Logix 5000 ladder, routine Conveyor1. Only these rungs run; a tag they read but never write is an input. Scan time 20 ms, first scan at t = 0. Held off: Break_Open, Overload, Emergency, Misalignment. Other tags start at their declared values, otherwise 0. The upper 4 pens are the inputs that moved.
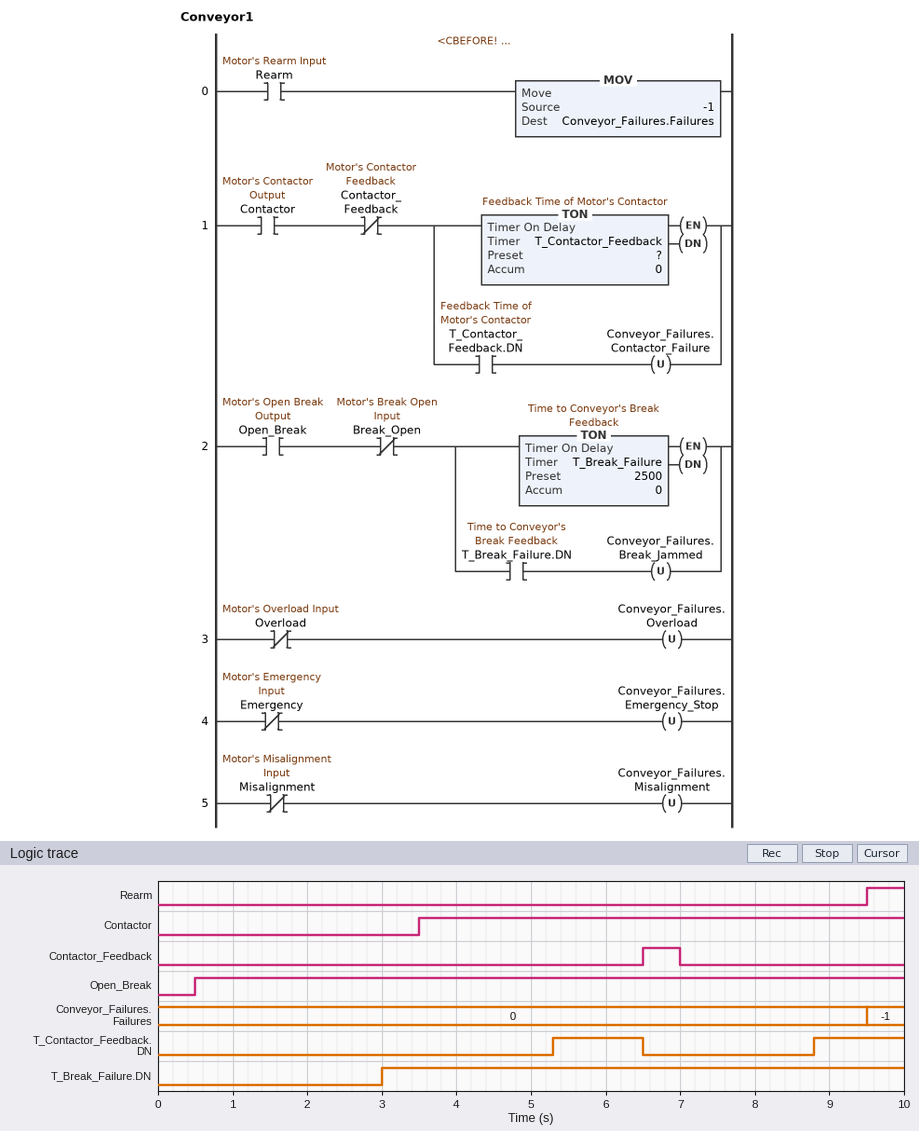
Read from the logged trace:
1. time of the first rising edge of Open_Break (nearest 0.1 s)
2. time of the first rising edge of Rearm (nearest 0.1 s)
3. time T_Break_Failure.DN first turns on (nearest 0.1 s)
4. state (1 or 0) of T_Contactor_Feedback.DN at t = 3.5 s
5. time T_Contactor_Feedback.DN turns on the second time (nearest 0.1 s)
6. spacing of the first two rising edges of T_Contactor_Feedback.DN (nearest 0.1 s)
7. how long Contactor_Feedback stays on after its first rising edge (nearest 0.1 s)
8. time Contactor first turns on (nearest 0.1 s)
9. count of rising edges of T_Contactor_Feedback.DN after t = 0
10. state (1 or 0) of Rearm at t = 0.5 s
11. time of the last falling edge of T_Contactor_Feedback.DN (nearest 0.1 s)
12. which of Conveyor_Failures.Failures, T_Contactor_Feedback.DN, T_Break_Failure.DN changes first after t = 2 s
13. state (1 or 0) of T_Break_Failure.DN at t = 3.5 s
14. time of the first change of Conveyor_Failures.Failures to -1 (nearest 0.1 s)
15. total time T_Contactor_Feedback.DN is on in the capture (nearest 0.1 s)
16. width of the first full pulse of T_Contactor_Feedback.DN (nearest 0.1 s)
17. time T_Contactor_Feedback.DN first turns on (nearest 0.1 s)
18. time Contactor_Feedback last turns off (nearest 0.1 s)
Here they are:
0.5 s
9.5 s
3.0 s
0
8.8 s
3.5 s
0.5 s
3.5 s
2
0
6.5 s
T_Break_Failure.DN
1
9.5 s
2.4 s
1.2 s
5.3 s
7.0 s
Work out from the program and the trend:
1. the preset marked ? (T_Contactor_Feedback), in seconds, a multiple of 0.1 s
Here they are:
1.8 s
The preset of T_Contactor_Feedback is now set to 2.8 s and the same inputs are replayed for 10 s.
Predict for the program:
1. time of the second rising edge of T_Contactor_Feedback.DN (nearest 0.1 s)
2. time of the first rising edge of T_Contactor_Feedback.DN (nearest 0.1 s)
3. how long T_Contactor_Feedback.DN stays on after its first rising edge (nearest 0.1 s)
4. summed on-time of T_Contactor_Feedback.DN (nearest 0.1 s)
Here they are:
9.8 s
6.3 s
0.2 s
0.4 s
